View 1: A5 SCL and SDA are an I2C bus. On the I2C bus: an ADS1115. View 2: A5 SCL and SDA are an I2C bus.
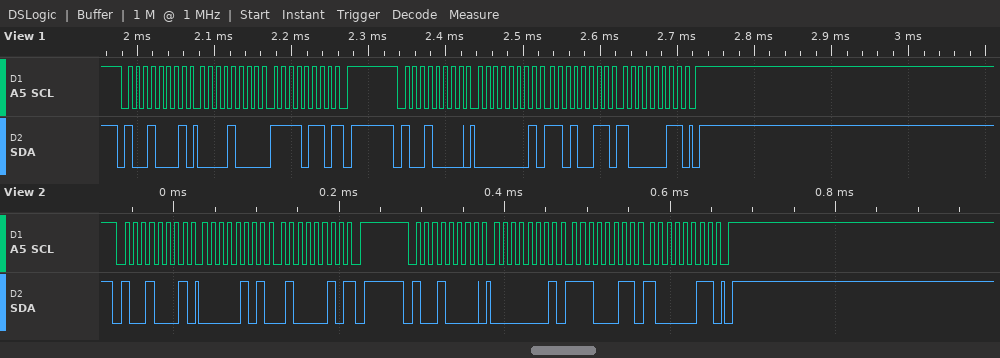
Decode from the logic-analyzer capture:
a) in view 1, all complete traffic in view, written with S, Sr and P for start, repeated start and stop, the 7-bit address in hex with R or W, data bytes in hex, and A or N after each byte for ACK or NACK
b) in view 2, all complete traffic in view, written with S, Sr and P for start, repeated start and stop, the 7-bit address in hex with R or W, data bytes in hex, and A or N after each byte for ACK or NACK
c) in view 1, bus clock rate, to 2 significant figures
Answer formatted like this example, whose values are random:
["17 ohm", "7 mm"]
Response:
["S 48R A 08 A F6 N P S 48W A 01 A D3 A 83 A P", "S 48R A 05 A 42 N P S 48W A 01 A E3 A 83 A P", "100 kHz"]
